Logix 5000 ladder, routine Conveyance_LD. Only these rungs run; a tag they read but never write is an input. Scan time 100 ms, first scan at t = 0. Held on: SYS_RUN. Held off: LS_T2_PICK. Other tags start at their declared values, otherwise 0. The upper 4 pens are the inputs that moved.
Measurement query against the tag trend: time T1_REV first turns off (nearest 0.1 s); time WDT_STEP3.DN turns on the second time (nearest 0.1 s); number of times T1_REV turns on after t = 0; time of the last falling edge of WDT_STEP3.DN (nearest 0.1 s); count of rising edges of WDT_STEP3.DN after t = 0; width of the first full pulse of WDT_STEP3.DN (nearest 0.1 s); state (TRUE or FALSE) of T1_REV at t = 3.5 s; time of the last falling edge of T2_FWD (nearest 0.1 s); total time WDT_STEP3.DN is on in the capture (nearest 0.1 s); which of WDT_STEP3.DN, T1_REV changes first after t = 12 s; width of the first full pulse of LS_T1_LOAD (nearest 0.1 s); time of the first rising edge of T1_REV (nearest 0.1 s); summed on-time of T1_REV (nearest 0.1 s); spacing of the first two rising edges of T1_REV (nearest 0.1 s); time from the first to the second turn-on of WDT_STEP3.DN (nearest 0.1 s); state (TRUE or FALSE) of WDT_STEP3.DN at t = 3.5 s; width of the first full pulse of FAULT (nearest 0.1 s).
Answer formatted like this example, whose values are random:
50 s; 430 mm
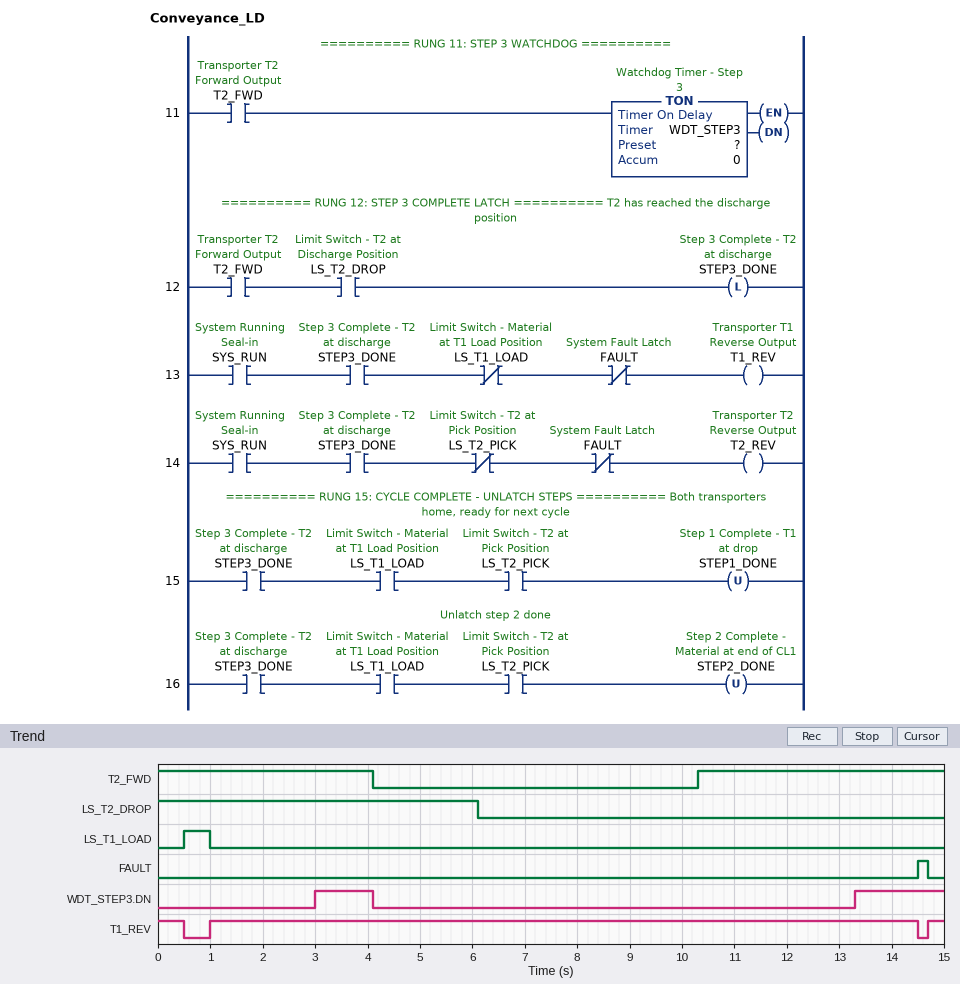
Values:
0.5 s; 13.3 s; 2; 4.1 s; 2; 1.1 s; TRUE; 4.1 s; 2.8 s; WDT_STEP3.DN; 0.5 s; 1.0 s; 14.3 s; 13.7 s; 10.3 s; TRUE; 0.2 s
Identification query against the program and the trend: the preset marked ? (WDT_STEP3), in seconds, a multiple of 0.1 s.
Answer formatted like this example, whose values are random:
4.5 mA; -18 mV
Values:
3.0 s
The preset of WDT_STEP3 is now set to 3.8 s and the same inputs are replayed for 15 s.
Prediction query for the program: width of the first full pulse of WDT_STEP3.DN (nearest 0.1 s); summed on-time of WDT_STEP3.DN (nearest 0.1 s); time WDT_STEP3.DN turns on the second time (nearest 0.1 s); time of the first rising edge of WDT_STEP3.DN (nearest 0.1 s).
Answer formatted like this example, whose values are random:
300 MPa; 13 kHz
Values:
0.3 s; 1.2 s; 14.1 s; 3.8 s
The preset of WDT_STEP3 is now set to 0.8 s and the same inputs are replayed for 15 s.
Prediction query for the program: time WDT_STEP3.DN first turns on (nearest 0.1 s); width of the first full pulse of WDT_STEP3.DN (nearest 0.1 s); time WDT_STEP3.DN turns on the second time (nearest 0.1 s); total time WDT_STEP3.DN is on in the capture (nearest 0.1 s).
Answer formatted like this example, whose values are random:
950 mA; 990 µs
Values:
0.8 s; 3.3 s; 11.1 s; 7.2 s
